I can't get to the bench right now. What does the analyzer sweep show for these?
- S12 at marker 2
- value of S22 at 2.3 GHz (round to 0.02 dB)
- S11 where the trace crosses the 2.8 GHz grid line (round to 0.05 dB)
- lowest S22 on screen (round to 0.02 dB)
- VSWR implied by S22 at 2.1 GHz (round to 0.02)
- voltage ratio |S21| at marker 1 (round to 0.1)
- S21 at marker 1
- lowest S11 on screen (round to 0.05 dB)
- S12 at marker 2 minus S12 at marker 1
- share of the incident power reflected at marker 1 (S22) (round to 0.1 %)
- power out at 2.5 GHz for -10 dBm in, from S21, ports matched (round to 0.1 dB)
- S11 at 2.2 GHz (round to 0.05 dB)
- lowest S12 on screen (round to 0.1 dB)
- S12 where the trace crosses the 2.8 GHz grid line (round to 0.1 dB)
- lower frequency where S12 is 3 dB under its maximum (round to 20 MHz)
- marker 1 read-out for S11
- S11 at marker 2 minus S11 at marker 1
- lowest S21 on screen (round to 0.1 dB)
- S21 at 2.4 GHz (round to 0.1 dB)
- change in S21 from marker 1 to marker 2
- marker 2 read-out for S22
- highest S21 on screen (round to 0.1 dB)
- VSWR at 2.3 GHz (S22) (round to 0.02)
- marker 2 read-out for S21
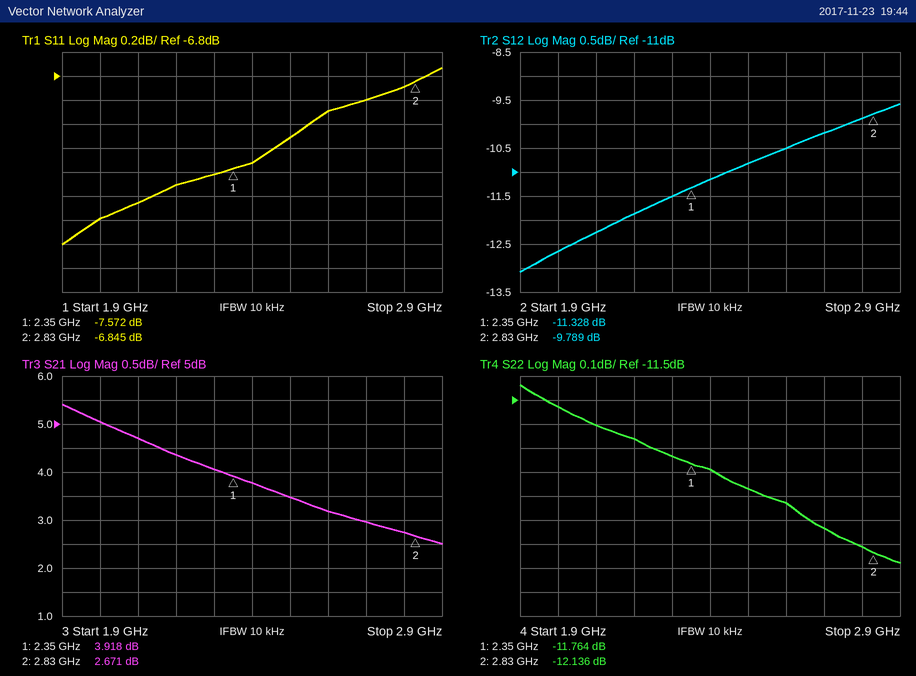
-9.789 dB
-11.74 dB
-6.90 dB
-12.18 dB
1.72
1.6
3.918 dB
-8.20 dB
1.539 dB
6.7 %
-6.5 dBm
-7.70 dB
-13.1 dB
-9.9 dB
2.02 GHz
-7.572 dB
0.727 dB
2.5 dB
3.8 dB
-1.247 dB
-12.136 dB
5.4 dB
1.70
2.671 dB
